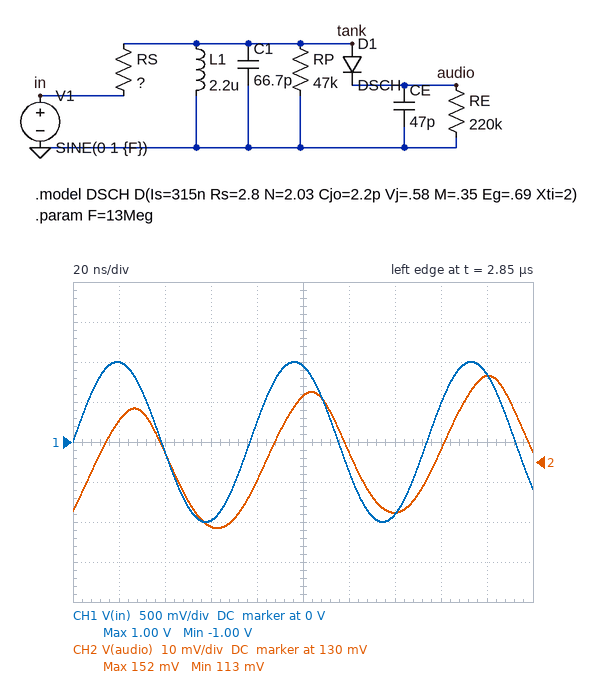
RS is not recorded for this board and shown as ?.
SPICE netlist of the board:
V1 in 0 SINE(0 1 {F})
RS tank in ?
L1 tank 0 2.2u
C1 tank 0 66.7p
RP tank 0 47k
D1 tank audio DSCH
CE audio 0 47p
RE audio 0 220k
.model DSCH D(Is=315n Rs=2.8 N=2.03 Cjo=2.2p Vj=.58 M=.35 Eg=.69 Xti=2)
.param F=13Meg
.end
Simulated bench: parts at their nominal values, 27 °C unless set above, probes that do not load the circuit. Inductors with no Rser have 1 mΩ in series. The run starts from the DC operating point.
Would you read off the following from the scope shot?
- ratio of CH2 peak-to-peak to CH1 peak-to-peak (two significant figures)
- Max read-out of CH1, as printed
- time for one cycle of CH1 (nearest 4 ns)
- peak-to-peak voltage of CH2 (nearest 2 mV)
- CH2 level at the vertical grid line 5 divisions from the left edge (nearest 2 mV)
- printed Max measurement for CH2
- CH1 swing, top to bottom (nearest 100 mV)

0.019
1.00 V
76 ns
38 mV
146 mV
152 mV
2.0 V
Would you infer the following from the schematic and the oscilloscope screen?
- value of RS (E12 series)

27 kΩ
